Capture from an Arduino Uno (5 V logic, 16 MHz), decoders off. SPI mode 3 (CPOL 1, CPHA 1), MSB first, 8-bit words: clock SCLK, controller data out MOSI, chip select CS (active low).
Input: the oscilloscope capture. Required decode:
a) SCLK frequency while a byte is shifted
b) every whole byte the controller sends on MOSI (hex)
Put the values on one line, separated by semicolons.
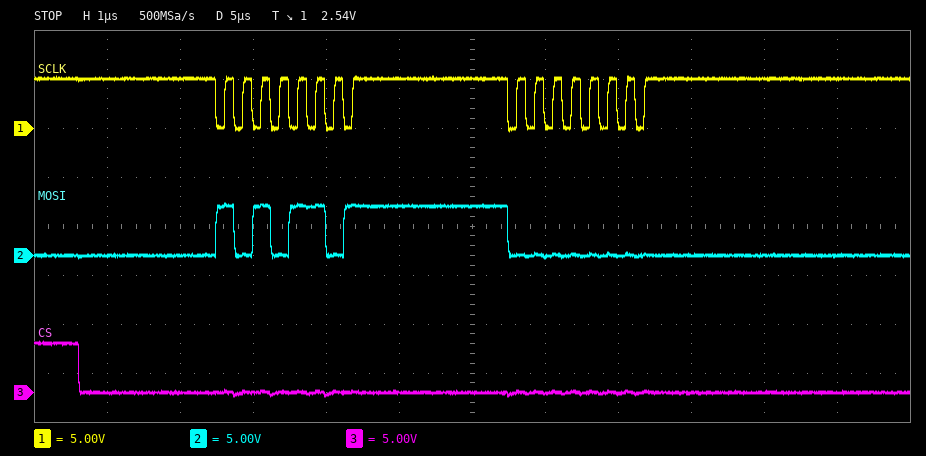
4 MHz; AD 00
